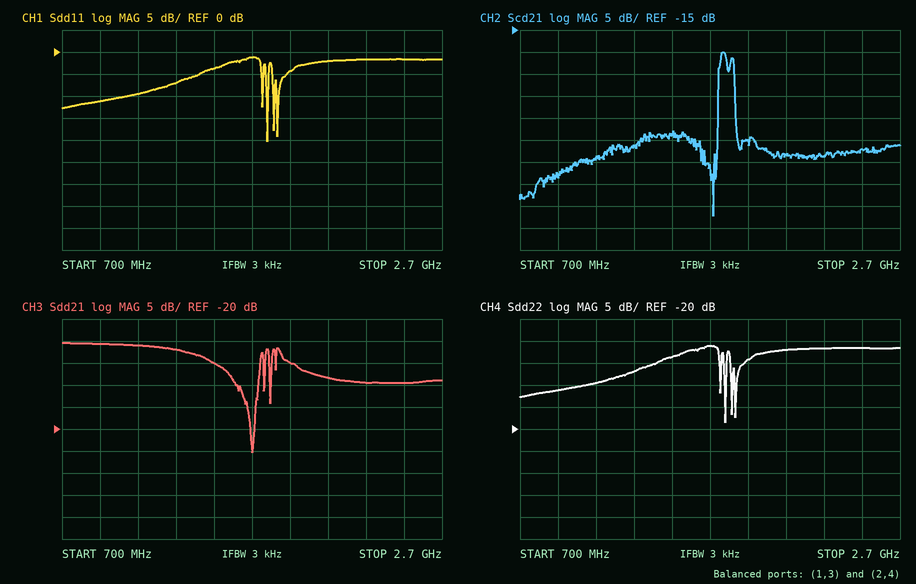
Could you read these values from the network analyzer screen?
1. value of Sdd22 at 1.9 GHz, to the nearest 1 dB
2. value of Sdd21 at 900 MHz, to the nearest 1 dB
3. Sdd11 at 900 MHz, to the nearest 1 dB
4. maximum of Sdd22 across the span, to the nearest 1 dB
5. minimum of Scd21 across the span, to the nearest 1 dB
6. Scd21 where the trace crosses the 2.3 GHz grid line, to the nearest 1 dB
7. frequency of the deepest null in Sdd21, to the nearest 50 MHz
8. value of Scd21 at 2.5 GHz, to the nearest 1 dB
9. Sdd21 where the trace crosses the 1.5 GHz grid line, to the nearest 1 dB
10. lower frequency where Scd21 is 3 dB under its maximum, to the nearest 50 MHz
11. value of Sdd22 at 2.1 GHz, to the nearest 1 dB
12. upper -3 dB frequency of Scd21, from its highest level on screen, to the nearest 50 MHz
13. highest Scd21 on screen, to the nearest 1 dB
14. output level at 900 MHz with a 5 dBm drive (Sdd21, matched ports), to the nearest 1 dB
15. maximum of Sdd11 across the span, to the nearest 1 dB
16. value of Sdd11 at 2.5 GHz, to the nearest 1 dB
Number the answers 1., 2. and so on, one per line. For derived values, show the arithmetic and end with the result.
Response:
1. -4 dB
2. -1 dB
3. -11 dB
4. -1 dB
5. -57 dB
6. -44 dB
7. 1.70 GHz
8. -42 dB
9. -5 dB
10. 1.75 GHz
11. -2 dB
12. 1.80 GHz
13. -20 dB
14. 5 dBm + (-1 dB) = 4 dBm
15. -1 dB
16. -2 dB
